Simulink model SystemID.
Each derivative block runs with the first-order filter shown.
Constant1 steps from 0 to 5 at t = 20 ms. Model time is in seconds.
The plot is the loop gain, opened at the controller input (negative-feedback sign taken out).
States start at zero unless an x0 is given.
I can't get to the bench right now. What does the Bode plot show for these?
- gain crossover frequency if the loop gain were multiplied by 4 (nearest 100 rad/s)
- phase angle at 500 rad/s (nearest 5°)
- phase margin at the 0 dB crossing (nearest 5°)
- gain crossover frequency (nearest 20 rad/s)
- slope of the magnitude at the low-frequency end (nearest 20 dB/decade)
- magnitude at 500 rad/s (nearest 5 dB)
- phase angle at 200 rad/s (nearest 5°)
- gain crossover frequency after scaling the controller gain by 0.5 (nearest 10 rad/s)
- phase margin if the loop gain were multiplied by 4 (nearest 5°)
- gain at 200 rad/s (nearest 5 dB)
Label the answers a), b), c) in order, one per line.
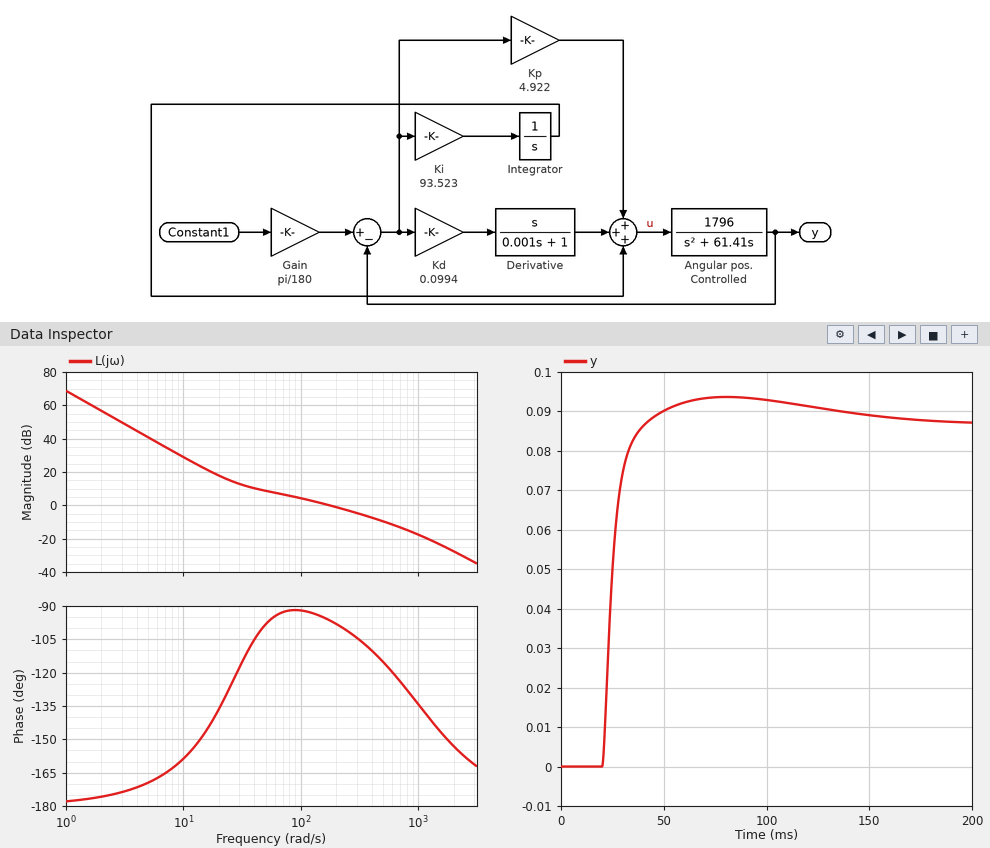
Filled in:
a) 600 rad/s
b) -115°
c) 85°
d) 180 rad/s
e) -40 dB/decade
f) -10 dB
g) -100°
h) 80 rad/s
i) 60°
j) 0 dB
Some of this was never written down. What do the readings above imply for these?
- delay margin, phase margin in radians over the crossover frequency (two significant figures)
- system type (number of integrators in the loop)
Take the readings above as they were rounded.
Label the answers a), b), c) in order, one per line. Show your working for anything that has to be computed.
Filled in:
a) 85 × π / 180 / 180 = 0.0082 s
b) 2
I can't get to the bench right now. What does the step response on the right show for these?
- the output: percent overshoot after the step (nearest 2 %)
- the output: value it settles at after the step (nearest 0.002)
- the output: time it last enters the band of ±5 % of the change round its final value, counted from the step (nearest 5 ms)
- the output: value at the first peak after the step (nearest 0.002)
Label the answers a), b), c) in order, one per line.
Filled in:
a) 8 %
b) 0.088
c) 95 ms
d) 0.094
